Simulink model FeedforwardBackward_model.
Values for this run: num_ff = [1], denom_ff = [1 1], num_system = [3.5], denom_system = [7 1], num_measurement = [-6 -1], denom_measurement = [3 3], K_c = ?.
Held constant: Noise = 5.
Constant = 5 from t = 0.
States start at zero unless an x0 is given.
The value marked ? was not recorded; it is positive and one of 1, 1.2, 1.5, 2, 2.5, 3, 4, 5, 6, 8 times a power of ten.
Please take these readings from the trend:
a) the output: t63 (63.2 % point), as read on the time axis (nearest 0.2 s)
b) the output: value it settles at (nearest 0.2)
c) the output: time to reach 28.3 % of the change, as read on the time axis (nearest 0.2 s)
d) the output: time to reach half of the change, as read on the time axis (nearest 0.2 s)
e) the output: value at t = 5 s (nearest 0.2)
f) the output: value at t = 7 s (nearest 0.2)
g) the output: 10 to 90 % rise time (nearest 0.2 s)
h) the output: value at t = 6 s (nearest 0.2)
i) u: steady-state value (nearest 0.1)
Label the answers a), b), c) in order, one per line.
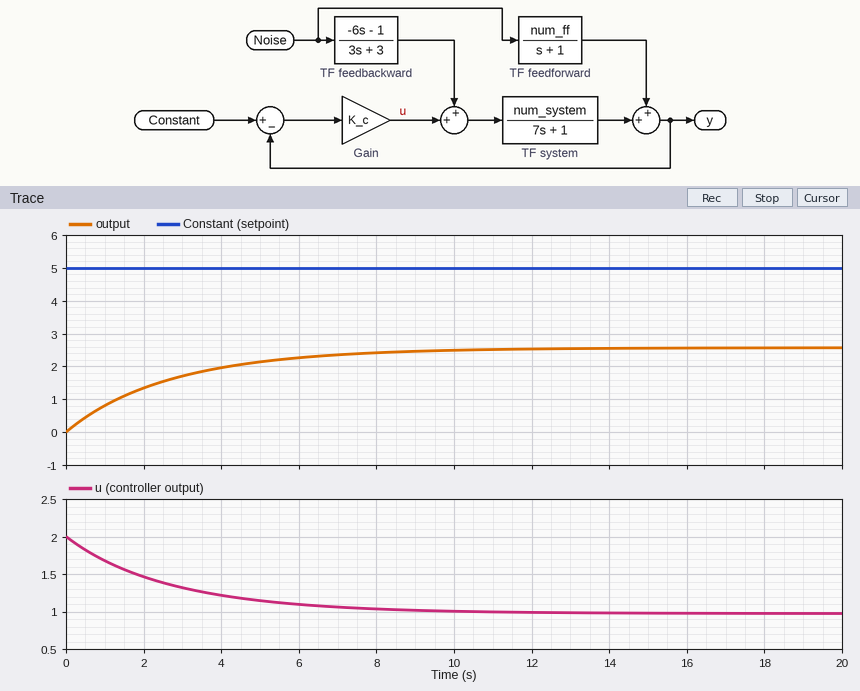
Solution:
a) 2.8 s
b) 2.6
c) 0.8 s
d) 1.8 s
e) 2.2
f) 2.4
g) 6.2 s
h) 2.2
i) 1.0
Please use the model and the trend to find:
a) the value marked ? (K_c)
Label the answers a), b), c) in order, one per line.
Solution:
a) 0.4
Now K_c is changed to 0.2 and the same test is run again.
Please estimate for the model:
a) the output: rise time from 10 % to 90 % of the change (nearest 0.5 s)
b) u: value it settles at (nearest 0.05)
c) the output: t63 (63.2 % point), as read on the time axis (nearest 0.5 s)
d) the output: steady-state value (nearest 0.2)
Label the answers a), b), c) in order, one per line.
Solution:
a) 8.5 s
b) 0.70
c) 3.5 s
d) 1.6
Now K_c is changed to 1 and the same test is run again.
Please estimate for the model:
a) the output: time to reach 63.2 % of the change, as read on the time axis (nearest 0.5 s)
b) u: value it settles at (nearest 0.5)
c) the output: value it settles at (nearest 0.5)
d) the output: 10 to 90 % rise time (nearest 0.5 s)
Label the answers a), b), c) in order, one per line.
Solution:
a) 1.5 s
b) 1.5
c) 3.5
d) 3.5 s
